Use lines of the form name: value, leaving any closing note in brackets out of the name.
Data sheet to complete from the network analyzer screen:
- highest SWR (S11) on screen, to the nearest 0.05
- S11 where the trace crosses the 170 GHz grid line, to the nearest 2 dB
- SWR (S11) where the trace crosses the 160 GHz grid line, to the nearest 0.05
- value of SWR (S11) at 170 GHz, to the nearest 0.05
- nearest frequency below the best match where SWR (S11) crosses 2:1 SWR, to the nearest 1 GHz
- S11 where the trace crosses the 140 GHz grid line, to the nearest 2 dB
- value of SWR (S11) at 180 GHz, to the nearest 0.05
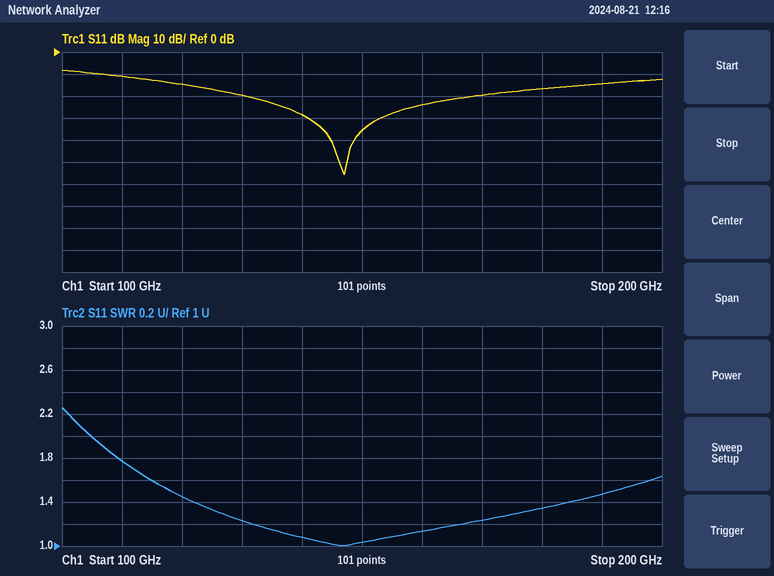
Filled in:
highest SWR (S11) on screen, to the nearest 0.05: 2.25
S11 where the trace crosses the 170 GHz grid line, to the nearest 2 dB: -20 dB
SWR (S11) where the trace crosses the 160 GHz grid line, to the nearest 0.05: 1.15
value of SWR (S11) at 170 GHz, to the nearest 0.05: 1.25
nearest frequency below the best match where SWR (S11) crosses 2:1 SWR, to the nearest 1 GHz: 105 GHz
S11 where the trace crosses the 140 GHz grid line, to the nearest 2 dB: -28 dB
value of SWR (S11) at 180 GHz, to the nearest 0.05: 1.35
